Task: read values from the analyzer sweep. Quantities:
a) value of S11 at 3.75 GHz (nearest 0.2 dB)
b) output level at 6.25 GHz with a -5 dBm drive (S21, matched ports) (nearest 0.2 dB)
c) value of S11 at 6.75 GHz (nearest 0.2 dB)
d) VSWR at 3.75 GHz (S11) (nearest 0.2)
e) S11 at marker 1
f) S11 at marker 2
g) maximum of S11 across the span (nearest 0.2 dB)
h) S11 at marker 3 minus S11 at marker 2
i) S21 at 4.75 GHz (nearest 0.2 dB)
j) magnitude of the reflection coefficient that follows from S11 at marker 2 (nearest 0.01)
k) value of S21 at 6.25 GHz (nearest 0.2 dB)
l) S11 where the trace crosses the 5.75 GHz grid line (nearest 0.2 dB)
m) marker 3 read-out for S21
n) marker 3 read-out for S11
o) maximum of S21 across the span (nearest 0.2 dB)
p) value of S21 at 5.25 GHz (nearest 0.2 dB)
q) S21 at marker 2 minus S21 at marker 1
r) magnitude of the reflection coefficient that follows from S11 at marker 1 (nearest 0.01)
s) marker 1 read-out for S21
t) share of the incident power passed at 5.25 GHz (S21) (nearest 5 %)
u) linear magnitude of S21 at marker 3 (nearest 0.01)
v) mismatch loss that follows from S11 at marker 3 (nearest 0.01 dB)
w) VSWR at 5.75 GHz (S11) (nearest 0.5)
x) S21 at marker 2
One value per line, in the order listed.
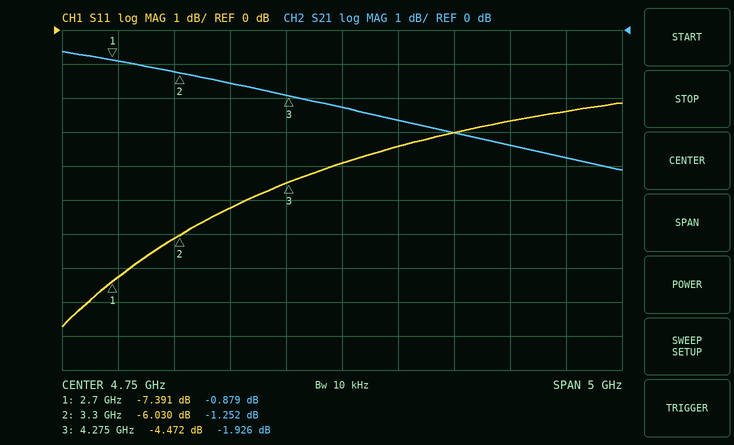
-5.2 dB
-8.4 dBm
-2.4 dB
3.4
-7.391 dB
-6.030 dB
-2.2 dB
1.558 dB
-2.2 dB
0.50
-3.4 dB
-3.0 dB
-1.926 dB
-4.472 dB
-0.6 dB
-2.6 dB
-0.373 dB
0.43
-0.879 dB
55 %
0.80
1.92 dB
6.0
-1.252 dB
